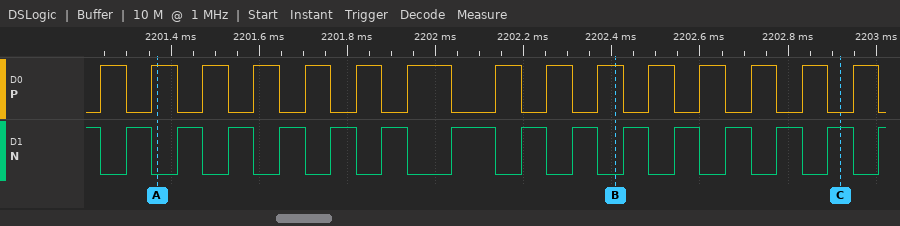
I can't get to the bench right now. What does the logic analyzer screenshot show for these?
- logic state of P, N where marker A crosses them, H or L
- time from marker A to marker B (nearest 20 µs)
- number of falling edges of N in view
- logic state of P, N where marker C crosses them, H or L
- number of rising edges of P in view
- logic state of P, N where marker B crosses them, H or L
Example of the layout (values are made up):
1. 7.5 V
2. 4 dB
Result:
1. P=H, N=L
2. 1040 µs
3. 15
4. P=L, N=H
5. 15
6. P=H, N=L
